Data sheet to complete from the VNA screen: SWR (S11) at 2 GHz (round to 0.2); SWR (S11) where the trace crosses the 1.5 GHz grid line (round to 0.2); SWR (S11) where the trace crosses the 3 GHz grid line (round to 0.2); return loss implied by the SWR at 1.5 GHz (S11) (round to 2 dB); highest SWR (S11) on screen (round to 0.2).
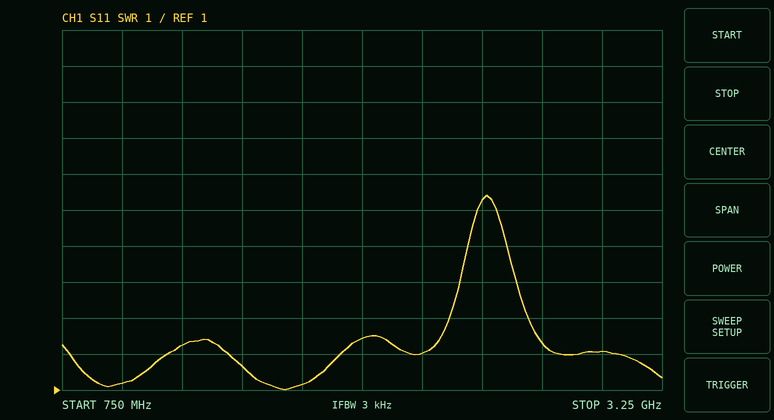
2.4
1.6
2.0
12 dB
6.4
